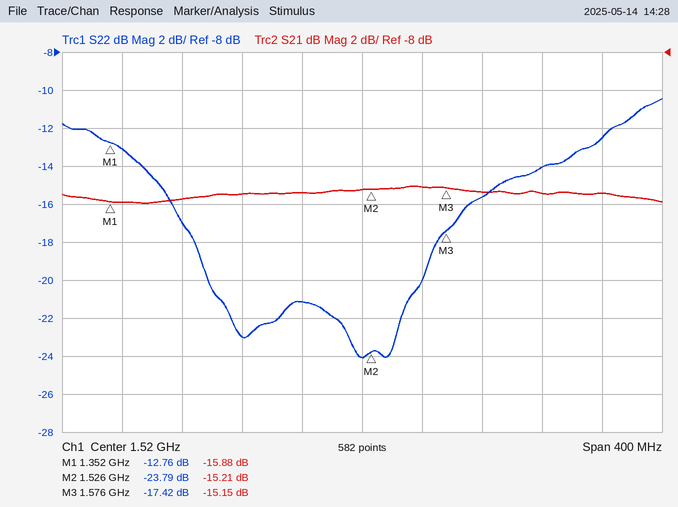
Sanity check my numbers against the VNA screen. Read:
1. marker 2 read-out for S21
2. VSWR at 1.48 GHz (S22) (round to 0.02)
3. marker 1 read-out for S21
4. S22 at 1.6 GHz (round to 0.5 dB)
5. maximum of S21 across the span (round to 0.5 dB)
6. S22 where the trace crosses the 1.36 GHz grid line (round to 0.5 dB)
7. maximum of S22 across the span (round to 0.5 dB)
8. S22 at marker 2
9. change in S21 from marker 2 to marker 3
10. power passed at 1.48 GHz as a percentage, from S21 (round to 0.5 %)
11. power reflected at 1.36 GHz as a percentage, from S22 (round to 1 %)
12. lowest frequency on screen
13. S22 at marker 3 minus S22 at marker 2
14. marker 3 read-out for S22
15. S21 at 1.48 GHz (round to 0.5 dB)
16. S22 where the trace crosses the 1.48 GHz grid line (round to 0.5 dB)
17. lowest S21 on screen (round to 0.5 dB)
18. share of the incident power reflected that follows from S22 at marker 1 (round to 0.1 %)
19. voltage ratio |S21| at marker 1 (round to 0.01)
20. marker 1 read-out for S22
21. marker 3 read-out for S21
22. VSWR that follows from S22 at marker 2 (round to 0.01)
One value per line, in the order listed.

-15.21 dB
1.20
-15.88 dB
-15.5 dB
-15.0 dB
-13.0 dB
-10.5 dB
-23.79 dB
0.06 dB
3.0 %
5 %
1.32 GHz
6.37 dB
-17.42 dB
-15.5 dB
-21.0 dB
-16.0 dB
5.3 %
0.16
-12.76 dB
-15.15 dB
1.14
